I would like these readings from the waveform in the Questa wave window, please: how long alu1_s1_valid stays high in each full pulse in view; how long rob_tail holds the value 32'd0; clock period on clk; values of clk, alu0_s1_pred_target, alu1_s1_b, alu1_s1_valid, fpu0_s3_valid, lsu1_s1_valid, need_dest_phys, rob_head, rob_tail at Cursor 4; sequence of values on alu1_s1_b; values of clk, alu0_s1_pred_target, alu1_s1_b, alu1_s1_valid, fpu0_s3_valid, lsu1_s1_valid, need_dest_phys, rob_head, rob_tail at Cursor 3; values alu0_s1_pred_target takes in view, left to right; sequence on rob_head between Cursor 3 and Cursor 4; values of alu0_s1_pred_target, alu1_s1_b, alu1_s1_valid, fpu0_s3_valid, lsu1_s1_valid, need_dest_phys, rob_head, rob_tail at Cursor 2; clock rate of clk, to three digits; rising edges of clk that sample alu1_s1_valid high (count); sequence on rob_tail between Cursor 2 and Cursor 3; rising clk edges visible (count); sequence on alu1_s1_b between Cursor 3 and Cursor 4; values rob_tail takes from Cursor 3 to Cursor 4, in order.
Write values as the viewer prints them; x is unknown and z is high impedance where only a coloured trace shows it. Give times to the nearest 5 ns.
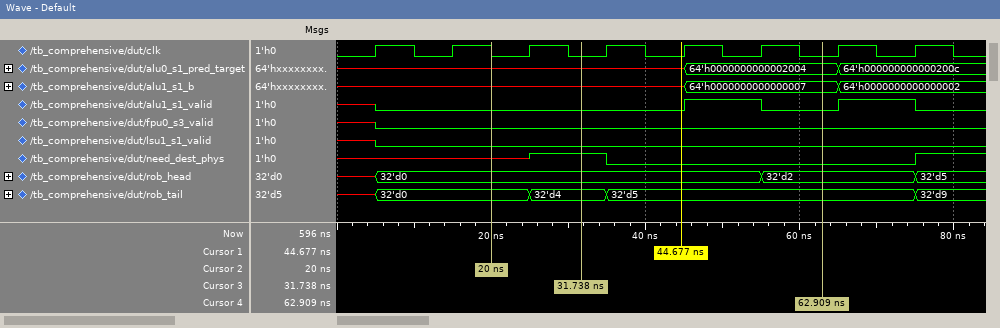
10 ns, 10 ns
20 ns
10 ns
clk=0, alu0_s1_pred_target=64'h0000000000002004, alu1_s1_b=64'h0000000000000007, alu1_s1_valid=0, fpu0_s3_valid=0, lsu1_s1_valid=0, need_dest_phys=0, rob_head=32'd2, rob_tail=32'd5
x, 64'h0000000000000007, 64'h0000000000000002
clk=0, alu0_s1_pred_target=x, alu1_s1_b=x, alu1_s1_valid=0, fpu0_s3_valid=0, lsu1_s1_valid=0, need_dest_phys=1, rob_head=32'd0, rob_tail=32'd4
x, 64'h0000000000002004, 64'h000000000000200c
32'd0, 32'd2
alu0_s1_pred_target=x, alu1_s1_b=x, alu1_s1_valid=0, fpu0_s3_valid=0, lsu1_s1_valid=0, need_dest_phys=x, rob_head=32'd0, rob_tail=32'd0
100 MHz
2
32'd0, 32'd4
8
x, 64'h0000000000000007
32'd4, 32'd5
